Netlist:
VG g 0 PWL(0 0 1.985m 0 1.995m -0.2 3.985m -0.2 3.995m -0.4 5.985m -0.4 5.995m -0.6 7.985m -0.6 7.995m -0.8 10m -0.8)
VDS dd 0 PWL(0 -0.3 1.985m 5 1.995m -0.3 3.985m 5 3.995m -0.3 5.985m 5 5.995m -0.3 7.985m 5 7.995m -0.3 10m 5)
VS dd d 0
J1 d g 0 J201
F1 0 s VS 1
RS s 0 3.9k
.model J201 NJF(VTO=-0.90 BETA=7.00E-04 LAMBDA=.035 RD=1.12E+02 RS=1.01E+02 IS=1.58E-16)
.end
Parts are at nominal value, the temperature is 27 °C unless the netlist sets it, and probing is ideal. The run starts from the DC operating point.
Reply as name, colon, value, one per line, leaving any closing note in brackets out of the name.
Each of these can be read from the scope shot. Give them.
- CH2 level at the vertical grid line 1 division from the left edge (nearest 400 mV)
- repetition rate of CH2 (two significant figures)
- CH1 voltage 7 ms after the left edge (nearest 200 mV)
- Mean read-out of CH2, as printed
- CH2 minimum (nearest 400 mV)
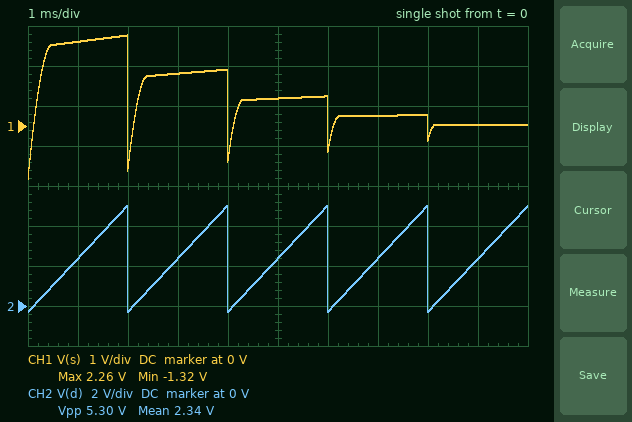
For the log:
CH2 level at the vertical grid line 1 division from the left edge: 2.4 V
repetition rate of CH2: 500 Hz
CH1 voltage 7 ms after the left edge: 200 mV
Mean read-out of CH2, as printed: 2.34 V
CH2 minimum: -400 mV
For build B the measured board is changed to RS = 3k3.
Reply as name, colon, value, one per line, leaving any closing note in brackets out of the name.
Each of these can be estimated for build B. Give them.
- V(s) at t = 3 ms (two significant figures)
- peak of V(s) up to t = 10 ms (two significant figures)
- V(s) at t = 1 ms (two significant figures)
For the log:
V(s) at t = 3 ms: 1.1 V
peak of V(s) up to t = 10 ms: 1.9 V
V(s) at t = 1 ms: 1.8 V
